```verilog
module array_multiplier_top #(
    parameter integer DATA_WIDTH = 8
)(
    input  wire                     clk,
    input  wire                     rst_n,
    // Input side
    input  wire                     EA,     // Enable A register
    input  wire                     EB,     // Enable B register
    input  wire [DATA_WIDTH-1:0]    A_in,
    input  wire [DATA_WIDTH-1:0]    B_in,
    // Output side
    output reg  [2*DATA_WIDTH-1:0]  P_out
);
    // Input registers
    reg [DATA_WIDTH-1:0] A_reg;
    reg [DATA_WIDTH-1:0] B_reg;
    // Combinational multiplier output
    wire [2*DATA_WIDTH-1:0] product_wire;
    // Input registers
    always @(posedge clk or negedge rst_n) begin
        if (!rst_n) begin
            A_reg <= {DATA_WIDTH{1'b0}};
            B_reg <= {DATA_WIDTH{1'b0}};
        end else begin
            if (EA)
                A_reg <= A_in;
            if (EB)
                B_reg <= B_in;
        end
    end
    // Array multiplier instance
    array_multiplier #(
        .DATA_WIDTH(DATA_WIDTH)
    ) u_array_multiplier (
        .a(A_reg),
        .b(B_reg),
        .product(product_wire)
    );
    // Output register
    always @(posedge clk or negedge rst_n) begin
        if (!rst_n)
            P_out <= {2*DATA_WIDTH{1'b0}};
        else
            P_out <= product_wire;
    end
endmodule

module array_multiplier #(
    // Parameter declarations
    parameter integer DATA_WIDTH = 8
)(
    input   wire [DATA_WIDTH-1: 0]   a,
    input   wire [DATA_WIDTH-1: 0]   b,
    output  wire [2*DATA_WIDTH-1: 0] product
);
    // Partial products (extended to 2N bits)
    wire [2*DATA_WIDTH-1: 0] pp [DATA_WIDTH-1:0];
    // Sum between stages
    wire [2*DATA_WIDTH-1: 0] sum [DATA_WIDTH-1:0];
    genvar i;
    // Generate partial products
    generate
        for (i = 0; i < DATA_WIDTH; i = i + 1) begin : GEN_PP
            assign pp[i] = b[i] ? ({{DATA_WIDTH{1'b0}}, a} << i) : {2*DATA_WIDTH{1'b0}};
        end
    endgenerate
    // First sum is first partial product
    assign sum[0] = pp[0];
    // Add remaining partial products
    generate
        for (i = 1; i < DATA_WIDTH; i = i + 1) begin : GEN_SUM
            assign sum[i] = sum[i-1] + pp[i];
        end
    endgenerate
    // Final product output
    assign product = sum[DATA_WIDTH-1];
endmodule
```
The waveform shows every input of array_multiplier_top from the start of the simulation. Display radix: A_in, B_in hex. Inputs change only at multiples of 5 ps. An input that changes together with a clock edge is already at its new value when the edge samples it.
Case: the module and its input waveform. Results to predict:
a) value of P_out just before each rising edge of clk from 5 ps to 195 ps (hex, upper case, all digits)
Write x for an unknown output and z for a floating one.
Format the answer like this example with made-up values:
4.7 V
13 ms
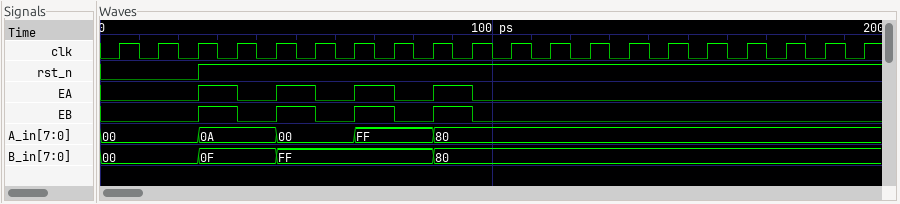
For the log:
0000, 0000, 0000, 0000, 0096, 0096, 0000, 0000, FE01, FE01, 4000, 4000, 4000, 4000, 4000, 4000, 4000, 4000, 4000, 4000
